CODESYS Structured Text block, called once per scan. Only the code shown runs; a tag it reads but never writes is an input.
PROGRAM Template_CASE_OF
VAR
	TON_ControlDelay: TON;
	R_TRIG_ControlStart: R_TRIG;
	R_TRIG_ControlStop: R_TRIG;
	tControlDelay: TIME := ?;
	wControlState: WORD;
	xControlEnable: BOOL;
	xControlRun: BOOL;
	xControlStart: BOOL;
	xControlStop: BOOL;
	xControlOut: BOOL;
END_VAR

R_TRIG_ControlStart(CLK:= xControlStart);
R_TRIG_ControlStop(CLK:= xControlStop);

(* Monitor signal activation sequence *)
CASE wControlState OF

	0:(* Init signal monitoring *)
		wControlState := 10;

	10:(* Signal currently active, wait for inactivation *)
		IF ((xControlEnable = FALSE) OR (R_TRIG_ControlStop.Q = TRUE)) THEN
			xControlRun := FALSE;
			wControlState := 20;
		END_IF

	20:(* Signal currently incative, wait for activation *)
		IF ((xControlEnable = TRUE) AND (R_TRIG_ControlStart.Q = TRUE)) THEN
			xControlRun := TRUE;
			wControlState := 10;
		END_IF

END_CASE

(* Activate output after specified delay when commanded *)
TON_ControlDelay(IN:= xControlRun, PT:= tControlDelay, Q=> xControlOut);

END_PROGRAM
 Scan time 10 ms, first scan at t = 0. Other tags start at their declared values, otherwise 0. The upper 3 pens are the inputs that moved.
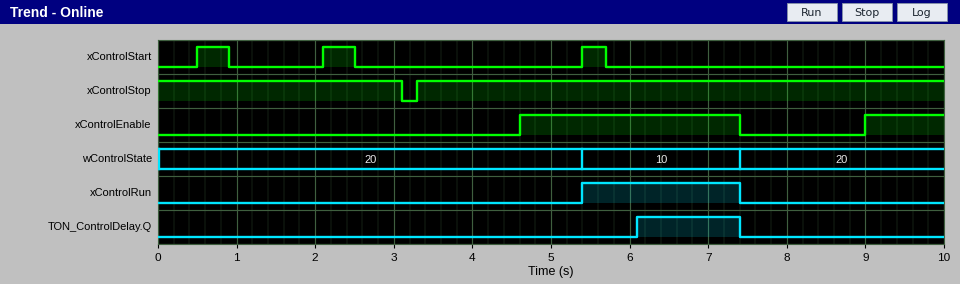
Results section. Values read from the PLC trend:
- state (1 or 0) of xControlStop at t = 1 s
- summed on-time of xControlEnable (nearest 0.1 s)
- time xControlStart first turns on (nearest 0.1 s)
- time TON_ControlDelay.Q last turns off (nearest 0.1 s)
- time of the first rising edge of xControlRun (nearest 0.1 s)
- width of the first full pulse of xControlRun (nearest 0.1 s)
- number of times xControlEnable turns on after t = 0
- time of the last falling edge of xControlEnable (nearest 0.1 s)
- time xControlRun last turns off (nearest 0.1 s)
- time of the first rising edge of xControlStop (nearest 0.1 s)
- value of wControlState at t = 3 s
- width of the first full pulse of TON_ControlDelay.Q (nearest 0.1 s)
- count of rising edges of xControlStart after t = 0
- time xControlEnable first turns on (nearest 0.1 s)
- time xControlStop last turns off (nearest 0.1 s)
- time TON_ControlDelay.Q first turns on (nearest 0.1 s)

1
3.8 s
0.5 s
7.4 s
5.4 s
2.0 s
2
7.4 s
7.4 s
3.3 s
20
1.3 s
3
4.6 s
3.1 s
6.1 s
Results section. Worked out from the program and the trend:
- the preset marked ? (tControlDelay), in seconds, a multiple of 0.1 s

0.7 s
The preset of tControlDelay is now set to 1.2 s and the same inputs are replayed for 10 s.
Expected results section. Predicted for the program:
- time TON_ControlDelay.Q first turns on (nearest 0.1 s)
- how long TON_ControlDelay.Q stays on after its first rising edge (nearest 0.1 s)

6.6 s
0.8 s
